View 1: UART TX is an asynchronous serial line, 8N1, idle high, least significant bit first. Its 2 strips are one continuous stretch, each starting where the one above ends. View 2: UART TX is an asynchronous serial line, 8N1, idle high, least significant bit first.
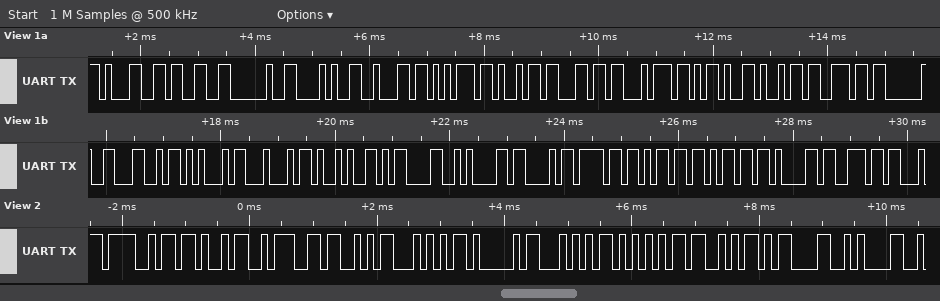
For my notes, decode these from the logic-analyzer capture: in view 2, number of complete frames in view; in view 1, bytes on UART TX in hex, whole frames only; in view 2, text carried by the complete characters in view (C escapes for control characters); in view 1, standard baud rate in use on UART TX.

11
31 33 20 28 62 75 69 6C 74 2D 69 6E 20 4C 45 44 29 0D 0A 43 6F 6D 6D 61 6E
"OK:STATUS\r\n"
9600 baud
